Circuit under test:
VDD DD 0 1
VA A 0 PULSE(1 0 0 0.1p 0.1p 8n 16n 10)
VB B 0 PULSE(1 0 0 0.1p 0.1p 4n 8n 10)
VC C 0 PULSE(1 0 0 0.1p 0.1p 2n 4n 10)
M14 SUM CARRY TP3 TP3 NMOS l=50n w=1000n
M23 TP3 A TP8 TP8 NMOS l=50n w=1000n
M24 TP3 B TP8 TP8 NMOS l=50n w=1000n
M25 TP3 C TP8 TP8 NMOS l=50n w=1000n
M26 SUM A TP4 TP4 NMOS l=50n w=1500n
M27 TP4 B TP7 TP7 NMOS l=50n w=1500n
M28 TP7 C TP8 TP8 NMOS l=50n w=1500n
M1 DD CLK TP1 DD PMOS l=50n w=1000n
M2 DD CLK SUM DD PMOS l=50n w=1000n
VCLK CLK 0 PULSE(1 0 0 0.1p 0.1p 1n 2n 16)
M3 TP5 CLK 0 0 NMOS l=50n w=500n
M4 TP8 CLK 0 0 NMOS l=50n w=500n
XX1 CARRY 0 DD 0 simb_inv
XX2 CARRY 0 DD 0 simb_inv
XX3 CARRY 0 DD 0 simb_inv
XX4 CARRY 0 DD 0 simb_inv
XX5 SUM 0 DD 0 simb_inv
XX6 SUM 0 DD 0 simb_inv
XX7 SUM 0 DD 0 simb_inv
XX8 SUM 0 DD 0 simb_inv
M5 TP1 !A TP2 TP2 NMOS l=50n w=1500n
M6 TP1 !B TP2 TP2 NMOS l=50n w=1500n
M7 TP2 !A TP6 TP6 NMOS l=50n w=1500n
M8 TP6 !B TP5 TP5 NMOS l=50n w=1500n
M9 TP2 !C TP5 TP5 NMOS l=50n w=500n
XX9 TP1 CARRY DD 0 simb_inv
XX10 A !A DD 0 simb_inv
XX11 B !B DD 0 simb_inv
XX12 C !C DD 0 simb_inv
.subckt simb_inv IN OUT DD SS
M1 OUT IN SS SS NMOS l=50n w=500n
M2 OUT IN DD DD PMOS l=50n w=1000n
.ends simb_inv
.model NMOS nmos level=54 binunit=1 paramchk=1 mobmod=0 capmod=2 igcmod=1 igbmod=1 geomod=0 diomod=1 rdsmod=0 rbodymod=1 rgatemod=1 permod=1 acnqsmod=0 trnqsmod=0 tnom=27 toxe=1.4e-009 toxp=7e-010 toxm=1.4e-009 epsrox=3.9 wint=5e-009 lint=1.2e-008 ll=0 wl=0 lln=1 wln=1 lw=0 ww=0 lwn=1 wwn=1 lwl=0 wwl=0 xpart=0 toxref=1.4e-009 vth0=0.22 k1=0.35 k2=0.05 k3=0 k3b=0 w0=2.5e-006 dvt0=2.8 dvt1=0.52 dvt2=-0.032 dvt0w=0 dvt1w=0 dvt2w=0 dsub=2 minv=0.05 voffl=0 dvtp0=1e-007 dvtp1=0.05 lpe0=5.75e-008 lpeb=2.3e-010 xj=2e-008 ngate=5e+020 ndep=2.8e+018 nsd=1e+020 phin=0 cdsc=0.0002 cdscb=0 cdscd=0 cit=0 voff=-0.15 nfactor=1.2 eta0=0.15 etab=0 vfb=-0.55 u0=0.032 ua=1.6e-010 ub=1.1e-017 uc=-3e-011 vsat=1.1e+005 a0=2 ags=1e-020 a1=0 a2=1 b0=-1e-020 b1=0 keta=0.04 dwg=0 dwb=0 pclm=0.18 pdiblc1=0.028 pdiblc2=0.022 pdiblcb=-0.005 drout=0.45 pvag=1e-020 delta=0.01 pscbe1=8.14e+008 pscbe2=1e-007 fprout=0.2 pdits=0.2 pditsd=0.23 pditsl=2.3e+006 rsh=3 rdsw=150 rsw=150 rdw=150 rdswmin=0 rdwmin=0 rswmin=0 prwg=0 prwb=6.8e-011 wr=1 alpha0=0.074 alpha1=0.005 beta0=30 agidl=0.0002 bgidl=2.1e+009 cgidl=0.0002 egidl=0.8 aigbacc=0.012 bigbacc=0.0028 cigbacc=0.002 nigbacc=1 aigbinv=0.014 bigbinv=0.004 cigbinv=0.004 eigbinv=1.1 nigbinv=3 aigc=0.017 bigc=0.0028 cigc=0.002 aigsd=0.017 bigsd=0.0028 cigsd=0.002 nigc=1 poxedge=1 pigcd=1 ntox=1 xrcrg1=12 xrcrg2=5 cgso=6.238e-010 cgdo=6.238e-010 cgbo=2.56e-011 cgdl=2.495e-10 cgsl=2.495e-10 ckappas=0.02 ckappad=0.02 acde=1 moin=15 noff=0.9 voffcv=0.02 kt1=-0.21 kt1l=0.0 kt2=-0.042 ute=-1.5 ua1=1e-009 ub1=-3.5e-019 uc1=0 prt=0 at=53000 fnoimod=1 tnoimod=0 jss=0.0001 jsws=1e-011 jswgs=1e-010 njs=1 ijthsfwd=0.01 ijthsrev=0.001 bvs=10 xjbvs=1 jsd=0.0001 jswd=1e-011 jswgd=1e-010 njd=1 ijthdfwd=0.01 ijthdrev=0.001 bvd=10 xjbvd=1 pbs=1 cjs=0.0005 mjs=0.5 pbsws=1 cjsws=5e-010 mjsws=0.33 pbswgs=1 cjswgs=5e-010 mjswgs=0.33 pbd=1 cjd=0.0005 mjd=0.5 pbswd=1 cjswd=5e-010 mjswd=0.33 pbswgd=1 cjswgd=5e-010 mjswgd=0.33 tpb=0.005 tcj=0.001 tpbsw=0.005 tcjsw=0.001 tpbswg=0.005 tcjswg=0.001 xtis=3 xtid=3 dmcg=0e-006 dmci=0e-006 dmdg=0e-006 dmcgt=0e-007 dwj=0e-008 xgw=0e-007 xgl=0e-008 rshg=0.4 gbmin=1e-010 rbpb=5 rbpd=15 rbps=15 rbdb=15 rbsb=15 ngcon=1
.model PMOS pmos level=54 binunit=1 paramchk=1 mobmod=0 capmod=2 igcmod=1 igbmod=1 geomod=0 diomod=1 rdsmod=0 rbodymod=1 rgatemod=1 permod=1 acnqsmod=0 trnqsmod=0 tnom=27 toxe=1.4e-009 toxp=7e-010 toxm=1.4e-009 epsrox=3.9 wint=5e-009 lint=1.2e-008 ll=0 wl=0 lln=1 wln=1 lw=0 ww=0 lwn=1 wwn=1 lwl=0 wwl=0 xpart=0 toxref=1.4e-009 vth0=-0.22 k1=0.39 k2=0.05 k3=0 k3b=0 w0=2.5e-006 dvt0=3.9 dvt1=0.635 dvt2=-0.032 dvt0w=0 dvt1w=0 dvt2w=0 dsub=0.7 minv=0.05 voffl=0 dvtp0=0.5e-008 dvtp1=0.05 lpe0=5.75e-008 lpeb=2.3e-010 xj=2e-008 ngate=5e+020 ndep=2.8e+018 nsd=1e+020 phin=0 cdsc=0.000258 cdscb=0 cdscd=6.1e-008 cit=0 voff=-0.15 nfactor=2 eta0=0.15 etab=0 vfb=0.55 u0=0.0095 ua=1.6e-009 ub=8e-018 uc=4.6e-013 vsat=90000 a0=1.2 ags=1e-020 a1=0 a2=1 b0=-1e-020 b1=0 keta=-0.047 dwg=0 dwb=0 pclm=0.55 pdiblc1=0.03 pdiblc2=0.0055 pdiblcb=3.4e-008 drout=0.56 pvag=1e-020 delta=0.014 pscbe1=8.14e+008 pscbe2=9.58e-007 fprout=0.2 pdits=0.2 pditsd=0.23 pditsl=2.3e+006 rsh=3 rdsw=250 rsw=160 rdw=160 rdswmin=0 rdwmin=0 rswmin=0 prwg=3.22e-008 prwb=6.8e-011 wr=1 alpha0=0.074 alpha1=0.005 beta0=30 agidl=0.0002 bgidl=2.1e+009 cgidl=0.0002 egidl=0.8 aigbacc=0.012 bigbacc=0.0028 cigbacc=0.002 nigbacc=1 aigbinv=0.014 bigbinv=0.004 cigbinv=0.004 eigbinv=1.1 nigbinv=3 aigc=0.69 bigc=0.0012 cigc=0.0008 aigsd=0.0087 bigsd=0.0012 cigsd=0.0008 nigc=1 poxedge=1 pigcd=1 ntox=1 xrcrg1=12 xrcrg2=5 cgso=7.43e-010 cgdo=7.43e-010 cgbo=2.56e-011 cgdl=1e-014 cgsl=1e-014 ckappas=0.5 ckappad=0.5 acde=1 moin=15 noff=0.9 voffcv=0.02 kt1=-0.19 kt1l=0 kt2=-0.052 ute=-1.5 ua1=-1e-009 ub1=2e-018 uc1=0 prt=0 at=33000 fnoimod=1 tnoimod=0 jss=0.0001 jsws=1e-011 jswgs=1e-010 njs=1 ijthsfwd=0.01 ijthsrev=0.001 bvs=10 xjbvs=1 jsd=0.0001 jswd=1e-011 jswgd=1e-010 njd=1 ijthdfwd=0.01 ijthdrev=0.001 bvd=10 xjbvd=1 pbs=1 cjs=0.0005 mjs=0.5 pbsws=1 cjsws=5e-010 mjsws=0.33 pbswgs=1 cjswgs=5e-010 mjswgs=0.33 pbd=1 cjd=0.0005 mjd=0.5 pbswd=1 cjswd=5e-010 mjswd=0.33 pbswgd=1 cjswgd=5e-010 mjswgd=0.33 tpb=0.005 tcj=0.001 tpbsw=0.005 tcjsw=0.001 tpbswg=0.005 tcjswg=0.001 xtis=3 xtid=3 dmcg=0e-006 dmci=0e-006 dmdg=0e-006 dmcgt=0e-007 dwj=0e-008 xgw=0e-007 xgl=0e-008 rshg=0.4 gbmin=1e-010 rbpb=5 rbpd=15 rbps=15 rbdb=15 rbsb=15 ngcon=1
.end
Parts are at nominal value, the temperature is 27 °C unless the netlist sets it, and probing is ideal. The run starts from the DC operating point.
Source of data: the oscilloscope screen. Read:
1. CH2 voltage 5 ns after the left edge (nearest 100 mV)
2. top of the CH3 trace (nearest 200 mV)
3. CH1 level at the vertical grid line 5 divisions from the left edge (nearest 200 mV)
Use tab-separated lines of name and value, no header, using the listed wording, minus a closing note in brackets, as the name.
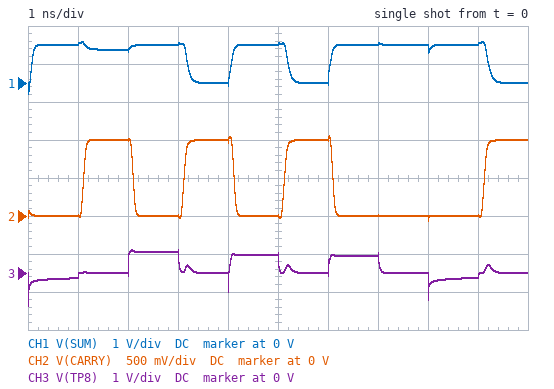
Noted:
CH2 voltage 5 ns after the left edge	0 V
top of the CH3 trace	600 mV
CH1 level at the vertical grid line 5 divisions from the left edge	1.0 V
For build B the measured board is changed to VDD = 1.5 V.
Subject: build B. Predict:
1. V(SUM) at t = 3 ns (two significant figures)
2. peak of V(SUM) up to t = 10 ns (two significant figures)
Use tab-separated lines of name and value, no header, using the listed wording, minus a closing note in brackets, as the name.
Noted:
V(SUM) at t = 3 ns	1.5 V
peak of V(SUM) up to t = 10 ns	1.6 V
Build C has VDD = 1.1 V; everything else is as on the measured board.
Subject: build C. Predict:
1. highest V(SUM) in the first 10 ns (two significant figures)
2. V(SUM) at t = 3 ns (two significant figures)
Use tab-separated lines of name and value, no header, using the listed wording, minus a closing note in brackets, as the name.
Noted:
highest V(SUM) in the first 10 ns	1.2 V
V(SUM) at t = 3 ns	1.1 V
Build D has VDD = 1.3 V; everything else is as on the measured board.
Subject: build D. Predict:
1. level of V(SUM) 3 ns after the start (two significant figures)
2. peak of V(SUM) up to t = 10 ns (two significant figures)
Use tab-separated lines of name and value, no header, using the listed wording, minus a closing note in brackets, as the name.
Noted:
level of V(SUM) 3 ns after the start	1.3 V
peak of V(SUM) up to t = 10 ns	1.4 V
